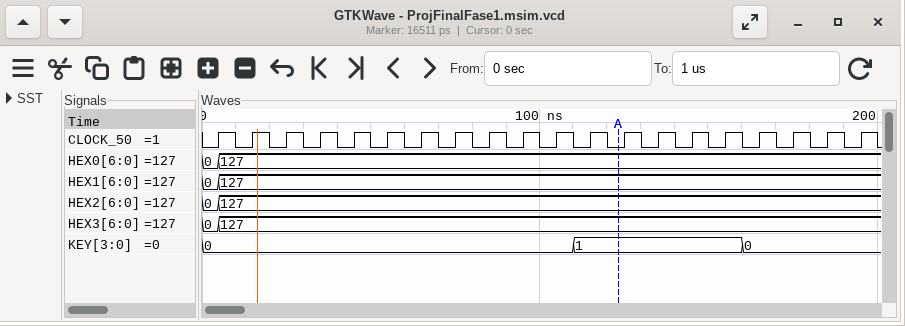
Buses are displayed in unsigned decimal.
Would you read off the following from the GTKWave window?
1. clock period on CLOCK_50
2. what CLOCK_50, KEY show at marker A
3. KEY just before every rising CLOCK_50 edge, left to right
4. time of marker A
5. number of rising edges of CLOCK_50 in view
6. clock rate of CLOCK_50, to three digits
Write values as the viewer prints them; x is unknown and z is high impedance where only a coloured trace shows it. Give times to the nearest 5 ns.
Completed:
10 ns
CLOCK_50=0, KEY=1
0, 0, 0, 0, 0, 0, 0, 0, 0, 0, 0, 1, 1, 1, 1, 1, 0, 0, 0, 0
125 ns
20
100 MHz
